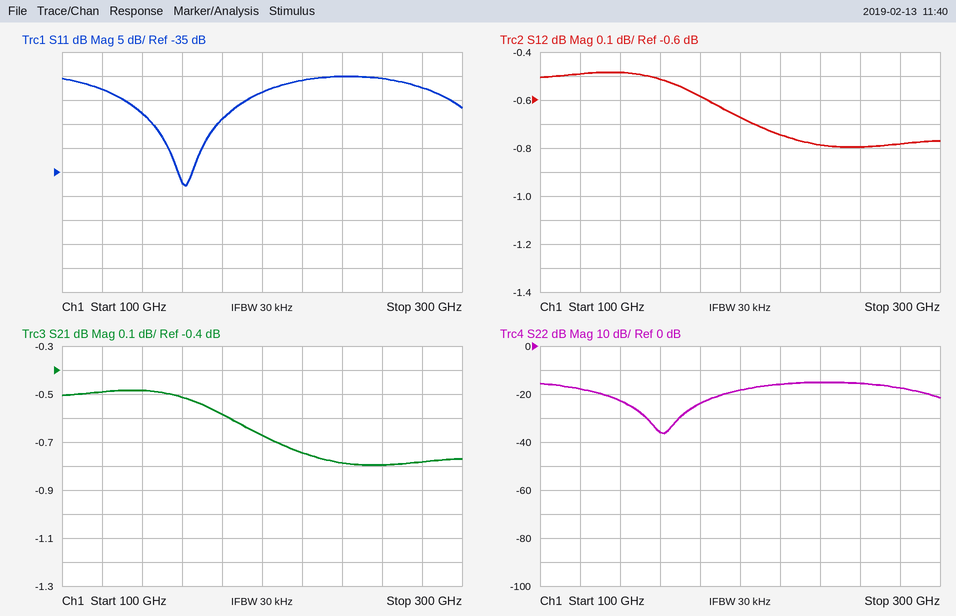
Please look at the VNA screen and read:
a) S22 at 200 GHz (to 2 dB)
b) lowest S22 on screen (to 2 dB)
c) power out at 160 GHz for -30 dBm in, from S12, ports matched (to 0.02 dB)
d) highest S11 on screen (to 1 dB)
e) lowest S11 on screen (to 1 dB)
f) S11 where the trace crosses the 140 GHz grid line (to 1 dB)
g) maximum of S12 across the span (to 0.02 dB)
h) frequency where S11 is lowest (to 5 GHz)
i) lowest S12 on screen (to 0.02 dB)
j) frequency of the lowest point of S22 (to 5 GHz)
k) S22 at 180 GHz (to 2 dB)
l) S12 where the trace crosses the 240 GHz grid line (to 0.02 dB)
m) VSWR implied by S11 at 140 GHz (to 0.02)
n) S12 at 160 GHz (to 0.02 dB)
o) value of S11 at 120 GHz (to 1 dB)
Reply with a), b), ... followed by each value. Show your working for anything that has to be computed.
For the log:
a) -18 dB
b) -36 dB
c) -30 dBm + (-0.52 dB) = -30.52 dBm
d) -15 dB
e) -38 dB
f) -23 dB
g) -0.48 dB
h) 160 GHz
i) -0.80 dB
j) 160 GHz
k) -24 dB
l) -0.78 dB
m) |Γ| = 10^(-23/20) = 0.0708; VSWR = (1 + 0.0708)/(1 − 0.0708) ≈ 1.15, so 1.16 to the nearest 0.02
n) -0.52 dB
o) -18 dB
